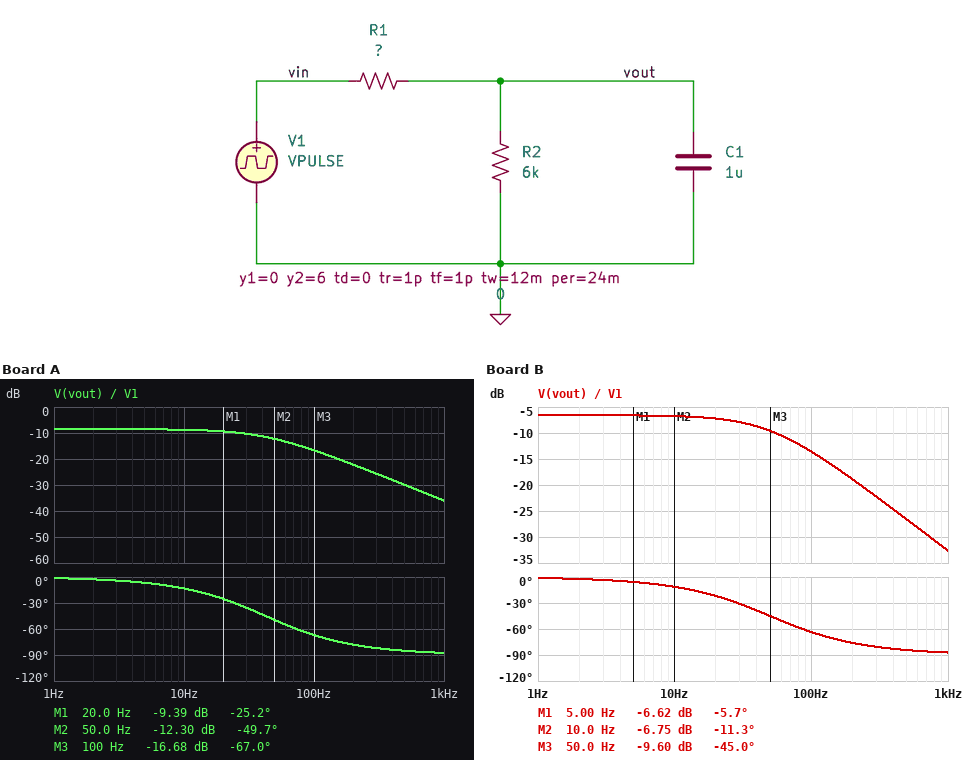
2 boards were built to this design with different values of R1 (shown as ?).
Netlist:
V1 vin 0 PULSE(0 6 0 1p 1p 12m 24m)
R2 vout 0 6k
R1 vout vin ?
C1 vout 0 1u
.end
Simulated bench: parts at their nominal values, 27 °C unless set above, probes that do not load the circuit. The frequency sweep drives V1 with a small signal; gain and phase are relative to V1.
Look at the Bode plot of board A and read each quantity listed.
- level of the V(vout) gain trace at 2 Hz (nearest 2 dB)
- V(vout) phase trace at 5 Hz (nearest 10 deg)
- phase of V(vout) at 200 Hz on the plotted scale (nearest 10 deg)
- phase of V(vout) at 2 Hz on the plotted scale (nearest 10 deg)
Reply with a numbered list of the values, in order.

1. -8 dB
2. -10 deg
3. -80 deg
4. 0 deg
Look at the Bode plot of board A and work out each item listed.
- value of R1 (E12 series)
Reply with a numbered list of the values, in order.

1. 10 kΩ
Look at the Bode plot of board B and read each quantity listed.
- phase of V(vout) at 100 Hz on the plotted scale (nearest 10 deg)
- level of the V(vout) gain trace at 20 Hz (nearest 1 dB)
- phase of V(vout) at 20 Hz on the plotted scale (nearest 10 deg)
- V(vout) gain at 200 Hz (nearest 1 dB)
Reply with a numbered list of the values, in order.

1. -60 deg
2. -7 dB
3. -20 deg
4. -19 dB
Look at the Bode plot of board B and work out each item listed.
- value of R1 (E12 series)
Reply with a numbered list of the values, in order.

1. 6.8 kΩ
